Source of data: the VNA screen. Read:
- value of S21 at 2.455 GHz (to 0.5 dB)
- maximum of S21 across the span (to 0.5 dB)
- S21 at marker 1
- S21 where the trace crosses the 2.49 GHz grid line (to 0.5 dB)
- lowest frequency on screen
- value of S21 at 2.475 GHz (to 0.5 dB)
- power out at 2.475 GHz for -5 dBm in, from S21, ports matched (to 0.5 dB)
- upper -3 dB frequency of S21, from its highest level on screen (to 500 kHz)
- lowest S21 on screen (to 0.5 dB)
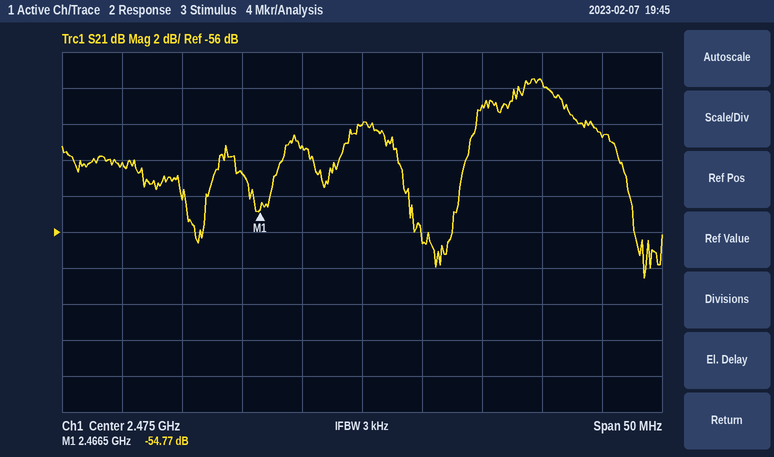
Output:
-52.0 dB
-47.5 dB
-54.77 dB
-47.5 dB
2.45 GHz
-50.0 dB
-55.0 dBm
2.4950 GHz
-58.5 dB
